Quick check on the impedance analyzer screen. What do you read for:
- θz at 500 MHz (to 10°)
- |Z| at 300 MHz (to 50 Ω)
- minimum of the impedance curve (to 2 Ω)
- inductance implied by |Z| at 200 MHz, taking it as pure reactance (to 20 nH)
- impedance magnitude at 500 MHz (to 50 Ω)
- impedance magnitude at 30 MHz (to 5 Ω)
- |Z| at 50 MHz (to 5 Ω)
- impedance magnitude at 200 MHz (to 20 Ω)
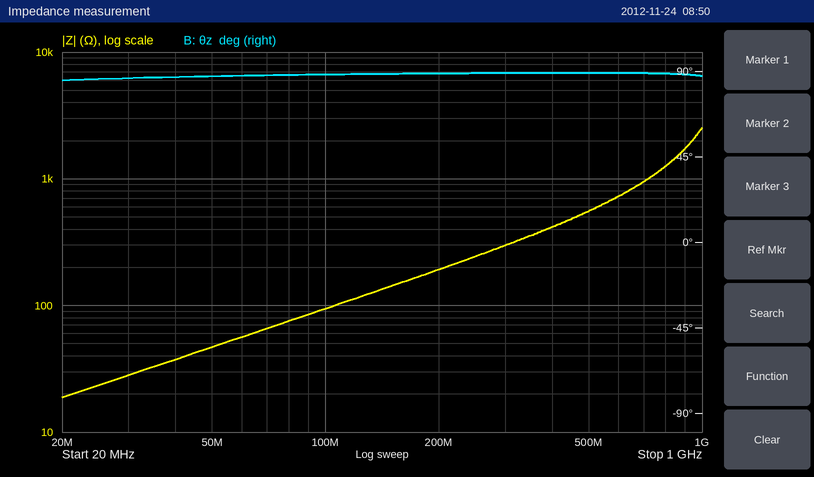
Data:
90°
300 Ω
18 Ω
160 nH
550 Ω
30 Ω
45 Ω
200 Ω
